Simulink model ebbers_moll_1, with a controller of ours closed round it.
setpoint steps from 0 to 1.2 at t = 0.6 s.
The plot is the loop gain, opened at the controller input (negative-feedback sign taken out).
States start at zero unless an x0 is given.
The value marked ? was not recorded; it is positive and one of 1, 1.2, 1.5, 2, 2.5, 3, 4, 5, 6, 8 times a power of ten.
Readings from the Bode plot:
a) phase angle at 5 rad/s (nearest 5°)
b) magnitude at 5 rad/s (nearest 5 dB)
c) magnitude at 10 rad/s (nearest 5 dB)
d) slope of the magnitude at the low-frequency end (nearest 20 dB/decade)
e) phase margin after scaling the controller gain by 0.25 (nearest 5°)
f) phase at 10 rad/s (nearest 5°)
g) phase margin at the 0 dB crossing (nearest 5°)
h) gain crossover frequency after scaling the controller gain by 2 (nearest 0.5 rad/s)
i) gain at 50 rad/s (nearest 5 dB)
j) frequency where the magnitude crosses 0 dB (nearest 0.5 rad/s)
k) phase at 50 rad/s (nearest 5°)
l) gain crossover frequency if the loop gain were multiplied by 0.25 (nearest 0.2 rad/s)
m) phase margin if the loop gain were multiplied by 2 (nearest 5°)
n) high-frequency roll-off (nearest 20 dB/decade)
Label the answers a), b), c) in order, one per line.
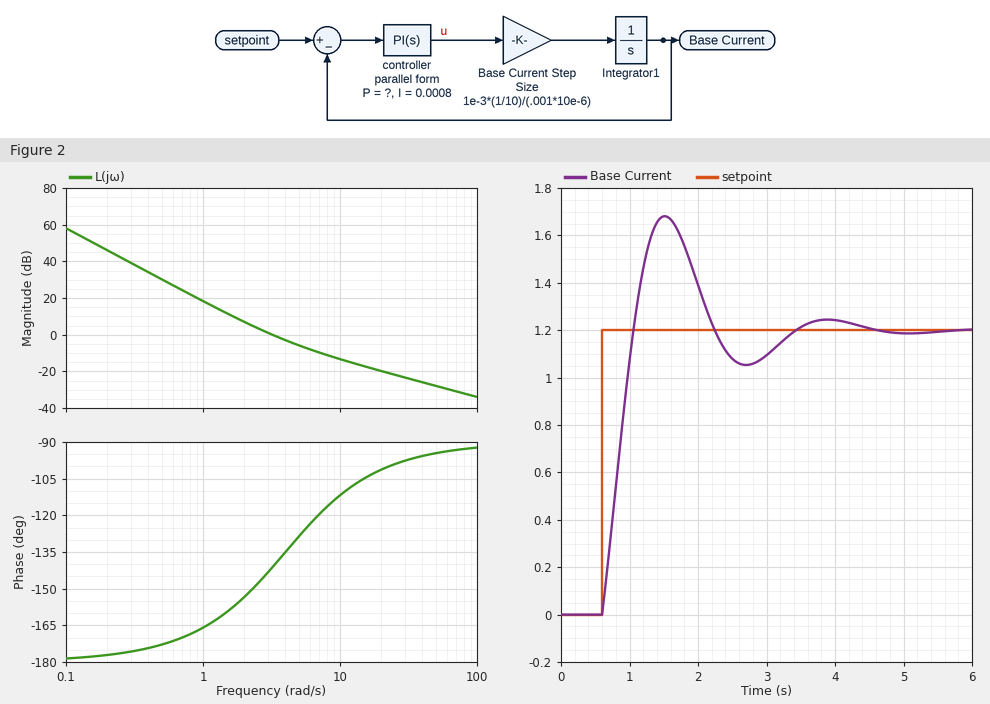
a) -130°
b) -5 dB
c) -15 dB
d) -40 dB/decade
e) 20°
f) -110°
g) 40°
h) 5.0 rad/s
i) -30 dB
j) 3.0 rad/s
k) -95°
l) 1.4 rad/s
m) 50°
n) -20 dB/decade
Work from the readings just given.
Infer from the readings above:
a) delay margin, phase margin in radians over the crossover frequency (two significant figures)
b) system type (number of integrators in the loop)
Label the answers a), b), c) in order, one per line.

a) 0.23 s
b) 2
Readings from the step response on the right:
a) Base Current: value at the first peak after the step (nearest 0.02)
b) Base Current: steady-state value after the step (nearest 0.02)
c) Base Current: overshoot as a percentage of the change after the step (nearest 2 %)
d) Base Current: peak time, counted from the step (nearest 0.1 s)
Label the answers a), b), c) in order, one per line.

a) 1.68
b) 1.20
c) 40 %
d) 0.9 s
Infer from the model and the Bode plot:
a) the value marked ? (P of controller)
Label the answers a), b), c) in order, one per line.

a) 0.0002
